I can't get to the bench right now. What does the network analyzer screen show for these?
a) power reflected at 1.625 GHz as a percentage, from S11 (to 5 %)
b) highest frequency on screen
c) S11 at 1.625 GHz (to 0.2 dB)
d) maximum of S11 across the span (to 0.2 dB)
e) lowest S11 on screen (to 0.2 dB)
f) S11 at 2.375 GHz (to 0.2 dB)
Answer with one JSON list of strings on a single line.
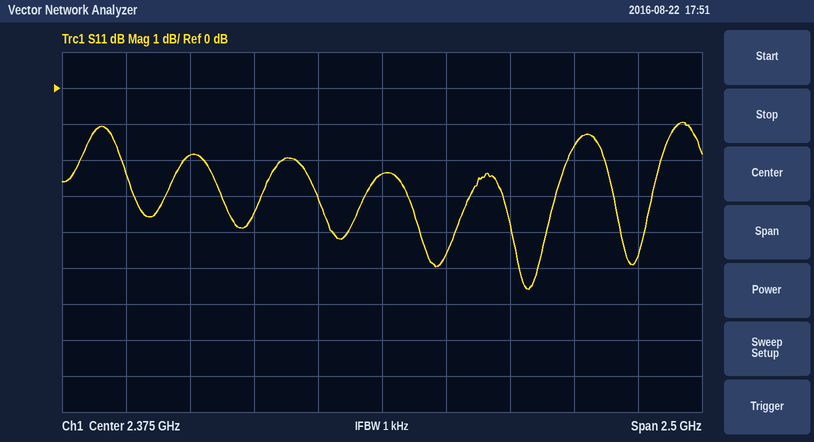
["65 %", "3.625 GHz", "-1.8 dB", "-1.0 dB", "-5.6 dB", "-2.4 dB"]
